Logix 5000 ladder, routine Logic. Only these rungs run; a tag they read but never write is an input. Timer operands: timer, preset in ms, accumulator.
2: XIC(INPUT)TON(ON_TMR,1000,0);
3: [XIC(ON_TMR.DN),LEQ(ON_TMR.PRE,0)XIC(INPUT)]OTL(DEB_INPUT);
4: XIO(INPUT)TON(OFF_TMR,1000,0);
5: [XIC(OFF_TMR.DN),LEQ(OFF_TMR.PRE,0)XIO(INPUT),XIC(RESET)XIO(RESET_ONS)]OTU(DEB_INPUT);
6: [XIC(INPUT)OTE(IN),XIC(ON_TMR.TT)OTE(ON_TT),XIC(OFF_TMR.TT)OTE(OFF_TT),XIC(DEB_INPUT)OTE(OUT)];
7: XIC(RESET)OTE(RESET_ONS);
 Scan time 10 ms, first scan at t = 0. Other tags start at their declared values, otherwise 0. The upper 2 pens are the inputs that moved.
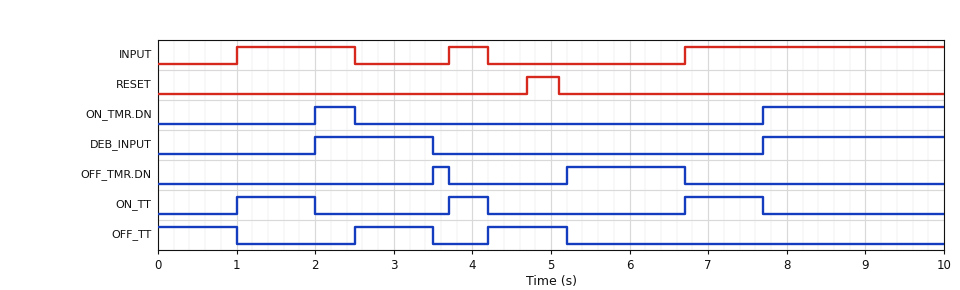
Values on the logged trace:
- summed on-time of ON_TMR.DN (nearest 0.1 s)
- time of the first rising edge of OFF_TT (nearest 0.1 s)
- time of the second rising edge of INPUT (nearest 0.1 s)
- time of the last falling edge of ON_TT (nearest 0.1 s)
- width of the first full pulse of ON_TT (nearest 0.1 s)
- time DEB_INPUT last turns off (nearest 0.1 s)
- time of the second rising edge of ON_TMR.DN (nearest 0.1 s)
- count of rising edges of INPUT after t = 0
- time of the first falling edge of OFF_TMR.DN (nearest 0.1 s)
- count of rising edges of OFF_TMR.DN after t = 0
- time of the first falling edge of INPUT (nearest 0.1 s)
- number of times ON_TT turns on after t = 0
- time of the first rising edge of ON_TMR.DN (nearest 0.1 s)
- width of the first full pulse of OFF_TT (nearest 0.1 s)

2.8 s
2.5 s
3.7 s
7.7 s
1.0 s
3.5 s
7.7 s
3
3.7 s
2
2.5 s
3
2.0 s
1.0 s
